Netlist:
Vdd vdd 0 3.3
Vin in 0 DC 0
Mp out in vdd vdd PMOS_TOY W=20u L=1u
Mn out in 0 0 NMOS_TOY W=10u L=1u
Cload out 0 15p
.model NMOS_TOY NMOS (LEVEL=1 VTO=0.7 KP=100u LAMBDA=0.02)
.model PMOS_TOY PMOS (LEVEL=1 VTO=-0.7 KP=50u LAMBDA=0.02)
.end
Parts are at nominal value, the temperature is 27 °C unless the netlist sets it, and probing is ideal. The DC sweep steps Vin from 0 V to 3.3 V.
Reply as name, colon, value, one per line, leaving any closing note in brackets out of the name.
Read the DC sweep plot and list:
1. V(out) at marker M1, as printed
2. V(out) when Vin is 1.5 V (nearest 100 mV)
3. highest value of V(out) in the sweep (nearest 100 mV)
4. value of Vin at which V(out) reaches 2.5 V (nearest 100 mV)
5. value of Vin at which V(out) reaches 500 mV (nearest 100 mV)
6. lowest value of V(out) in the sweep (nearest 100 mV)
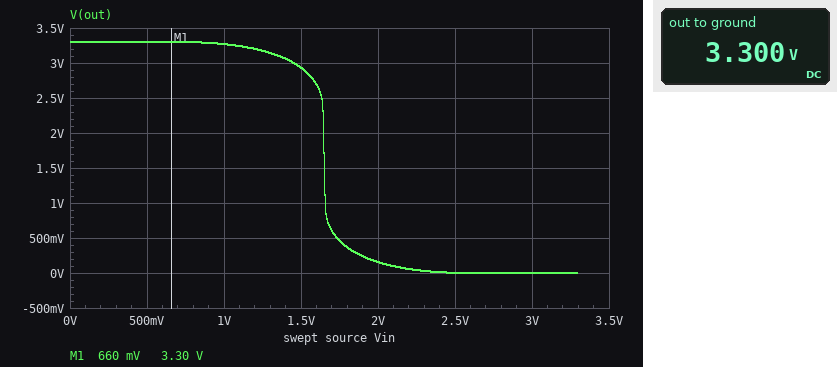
V(out) at marker M1, as printed: 3.30 V
V(out) when Vin is 1.5 V: 2.9 V
highest value of V(out) in the sweep: 3.3 V
value of Vin at which V(out) reaches 2.5 V: 1.6 V
value of Vin at which V(out) reaches 500 mV: 1.7 V
lowest value of V(out) in the sweep: 0 V
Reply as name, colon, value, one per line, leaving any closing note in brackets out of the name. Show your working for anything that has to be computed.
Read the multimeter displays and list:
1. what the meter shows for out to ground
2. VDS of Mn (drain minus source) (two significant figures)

what the meter shows for out to ground: 3.300 V
VDS of Mn (drain minus source): 3.3 V = 3.3 V
